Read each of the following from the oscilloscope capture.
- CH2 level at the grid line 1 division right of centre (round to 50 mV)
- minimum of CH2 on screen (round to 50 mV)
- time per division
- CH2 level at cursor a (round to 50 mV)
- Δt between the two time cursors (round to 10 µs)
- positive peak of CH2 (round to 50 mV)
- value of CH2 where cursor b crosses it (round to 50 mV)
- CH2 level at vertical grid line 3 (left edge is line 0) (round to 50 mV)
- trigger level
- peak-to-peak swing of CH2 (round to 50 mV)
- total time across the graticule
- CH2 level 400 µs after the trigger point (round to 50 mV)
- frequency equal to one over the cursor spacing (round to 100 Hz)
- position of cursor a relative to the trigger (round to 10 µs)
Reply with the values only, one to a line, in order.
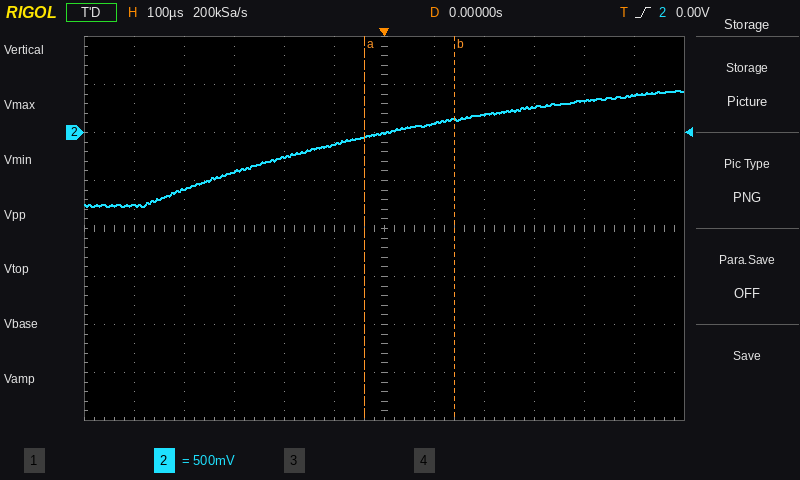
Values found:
100 mV
-750 mV
100 µs
-50 mV
180 µs
450 mV
150 mV
-400 mV
0.00 V
1.20 V
1.2 ms
350 mV
5.6 kHz
-40 µs
